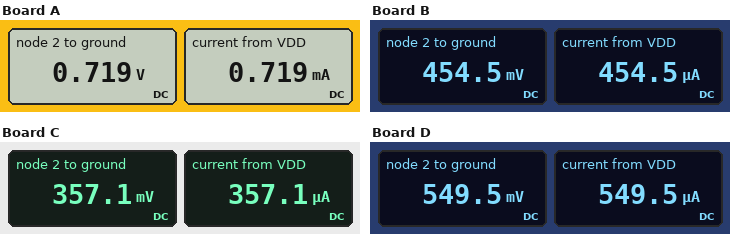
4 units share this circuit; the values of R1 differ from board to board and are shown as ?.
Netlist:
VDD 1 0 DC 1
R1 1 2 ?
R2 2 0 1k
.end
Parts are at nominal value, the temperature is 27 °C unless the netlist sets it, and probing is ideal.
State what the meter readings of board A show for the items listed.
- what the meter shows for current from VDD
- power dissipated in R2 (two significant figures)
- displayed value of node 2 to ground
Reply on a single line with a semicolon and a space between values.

0.719 mA; 520 µW; 0.719 V
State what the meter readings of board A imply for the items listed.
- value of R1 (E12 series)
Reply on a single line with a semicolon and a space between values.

390 Ω
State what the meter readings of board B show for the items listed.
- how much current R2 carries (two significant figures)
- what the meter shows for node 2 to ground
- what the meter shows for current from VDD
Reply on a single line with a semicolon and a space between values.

450 µA; 454.5 mV; 454.5 µA
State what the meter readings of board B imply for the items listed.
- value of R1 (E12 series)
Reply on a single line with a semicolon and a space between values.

1.2 kΩ
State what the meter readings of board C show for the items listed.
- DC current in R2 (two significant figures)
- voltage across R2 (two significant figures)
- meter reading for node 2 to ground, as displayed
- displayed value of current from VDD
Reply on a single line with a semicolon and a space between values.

360 µA; 360 mV; 357.1 mV; 357.1 µA
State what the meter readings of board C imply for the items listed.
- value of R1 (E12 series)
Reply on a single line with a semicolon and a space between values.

1.8 kΩ
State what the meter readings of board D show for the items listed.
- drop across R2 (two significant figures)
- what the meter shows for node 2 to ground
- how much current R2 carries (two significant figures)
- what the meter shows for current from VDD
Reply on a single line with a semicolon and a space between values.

550 mV; 549.5 mV; 550 µA; 549.5 µA
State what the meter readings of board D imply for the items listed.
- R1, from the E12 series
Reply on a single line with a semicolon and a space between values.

820 Ω
